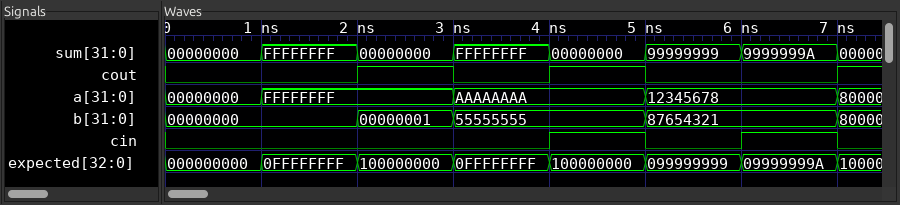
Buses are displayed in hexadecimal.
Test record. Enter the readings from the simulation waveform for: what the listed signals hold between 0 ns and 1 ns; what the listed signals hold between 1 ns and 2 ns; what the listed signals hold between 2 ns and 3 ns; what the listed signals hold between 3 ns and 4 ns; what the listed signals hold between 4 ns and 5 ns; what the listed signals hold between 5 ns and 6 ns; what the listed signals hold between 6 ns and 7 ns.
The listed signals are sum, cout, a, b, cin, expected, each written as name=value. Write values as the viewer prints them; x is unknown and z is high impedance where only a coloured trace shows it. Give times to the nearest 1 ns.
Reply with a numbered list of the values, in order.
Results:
1. sum=00000000, cout=0, a=00000000, b=00000000, cin=0, expected=000000000
2. sum=FFFFFFFF, cout=0, a=FFFFFFFF, b=00000000, cin=0, expected=0FFFFFFFF
3. sum=00000000, cout=1, a=FFFFFFFF, b=00000001, cin=0, expected=100000000
4. sum=FFFFFFFF, cout=0, a=AAAAAAAA, b=55555555, cin=0, expected=0FFFFFFFF
5. sum=00000000, cout=1, a=AAAAAAAA, b=55555555, cin=1, expected=100000000
6. sum=99999999, cout=0, a=12345678, b=87654321, cin=0, expected=099999999
7. sum=9999999A, cout=0, a=12345678, b=87654321, cin=1, expected=09999999A
